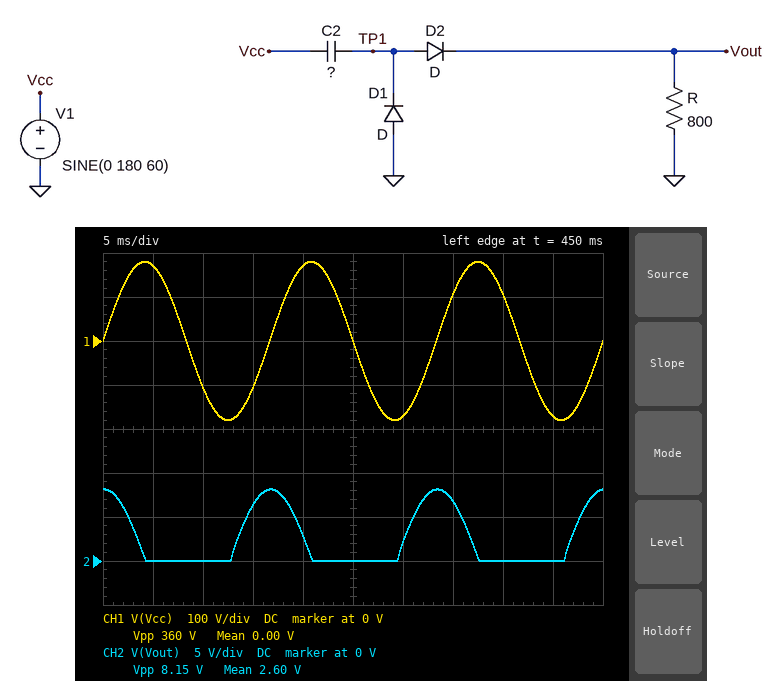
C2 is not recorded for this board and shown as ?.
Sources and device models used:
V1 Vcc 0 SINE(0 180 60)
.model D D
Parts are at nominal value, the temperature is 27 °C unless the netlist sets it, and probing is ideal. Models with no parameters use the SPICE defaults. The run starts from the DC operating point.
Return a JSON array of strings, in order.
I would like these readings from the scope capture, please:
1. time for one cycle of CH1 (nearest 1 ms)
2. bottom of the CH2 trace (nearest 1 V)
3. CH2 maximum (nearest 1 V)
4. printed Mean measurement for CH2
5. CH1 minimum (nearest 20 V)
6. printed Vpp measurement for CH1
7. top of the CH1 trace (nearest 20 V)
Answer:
["17 ms", "0 V", "8 V", "2.60 V", "-180 V", "360 V", "180 V"]
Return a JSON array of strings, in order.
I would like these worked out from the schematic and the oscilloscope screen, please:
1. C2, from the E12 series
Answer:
["150 nF"]
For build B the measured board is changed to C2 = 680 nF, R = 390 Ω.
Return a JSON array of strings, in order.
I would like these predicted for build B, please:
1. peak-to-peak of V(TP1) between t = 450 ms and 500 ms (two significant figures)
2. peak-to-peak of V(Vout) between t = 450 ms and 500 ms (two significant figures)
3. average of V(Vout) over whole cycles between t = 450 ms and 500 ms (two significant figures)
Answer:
["19 V", "18 V", "5.7 V"]
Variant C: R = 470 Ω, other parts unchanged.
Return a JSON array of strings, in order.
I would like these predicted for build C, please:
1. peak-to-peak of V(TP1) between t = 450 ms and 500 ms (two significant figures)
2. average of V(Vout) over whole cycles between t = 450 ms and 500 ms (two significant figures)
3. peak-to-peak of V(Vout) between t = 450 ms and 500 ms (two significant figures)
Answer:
["6.2 V", "1.5 V", "4.8 V"]
